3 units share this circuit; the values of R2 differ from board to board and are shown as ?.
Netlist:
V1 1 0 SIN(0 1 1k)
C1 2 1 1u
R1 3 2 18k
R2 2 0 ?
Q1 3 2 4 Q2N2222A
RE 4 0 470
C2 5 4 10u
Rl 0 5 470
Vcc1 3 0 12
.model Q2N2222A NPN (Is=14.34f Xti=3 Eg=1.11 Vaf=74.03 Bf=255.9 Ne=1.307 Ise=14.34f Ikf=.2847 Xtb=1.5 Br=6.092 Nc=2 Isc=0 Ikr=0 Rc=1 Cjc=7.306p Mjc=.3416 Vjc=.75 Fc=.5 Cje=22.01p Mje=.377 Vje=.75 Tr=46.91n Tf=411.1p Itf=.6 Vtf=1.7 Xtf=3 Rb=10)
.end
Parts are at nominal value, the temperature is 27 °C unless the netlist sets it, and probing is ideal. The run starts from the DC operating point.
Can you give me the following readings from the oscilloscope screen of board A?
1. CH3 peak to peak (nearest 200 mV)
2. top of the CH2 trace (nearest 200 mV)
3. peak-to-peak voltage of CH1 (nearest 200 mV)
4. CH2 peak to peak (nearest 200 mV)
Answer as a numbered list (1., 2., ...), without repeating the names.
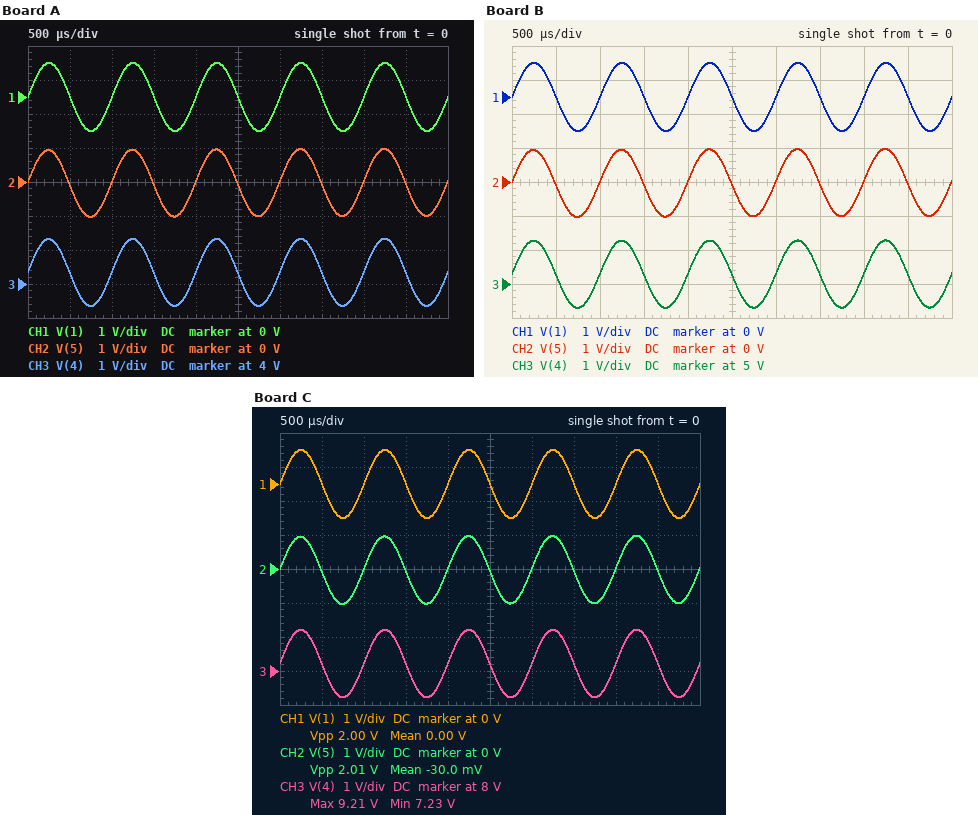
1. 2.0 V
2. 1.0 V
3. 2.0 V
4. 2.0 V
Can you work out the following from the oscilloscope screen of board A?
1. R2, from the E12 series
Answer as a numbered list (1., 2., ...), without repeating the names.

1. 15 kΩ
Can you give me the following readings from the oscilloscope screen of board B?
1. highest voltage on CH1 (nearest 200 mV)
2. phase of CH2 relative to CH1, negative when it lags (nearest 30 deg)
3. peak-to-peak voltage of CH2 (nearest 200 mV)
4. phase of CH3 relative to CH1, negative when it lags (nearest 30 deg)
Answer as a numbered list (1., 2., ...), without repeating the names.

1. 1.0 V
2. 0 deg
3. 2.0 V
4. 0 deg
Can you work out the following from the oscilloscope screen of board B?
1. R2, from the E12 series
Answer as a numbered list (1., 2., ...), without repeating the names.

1. 22 kΩ
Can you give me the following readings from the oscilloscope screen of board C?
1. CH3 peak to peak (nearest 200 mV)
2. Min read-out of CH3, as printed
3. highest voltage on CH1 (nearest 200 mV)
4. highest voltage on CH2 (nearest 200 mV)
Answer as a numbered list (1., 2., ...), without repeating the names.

1. 2.0 V
2. 7.23 V
3. 1.0 V
4. 1.0 V
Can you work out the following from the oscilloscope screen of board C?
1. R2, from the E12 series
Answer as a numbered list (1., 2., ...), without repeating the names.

1. 120 kΩ
